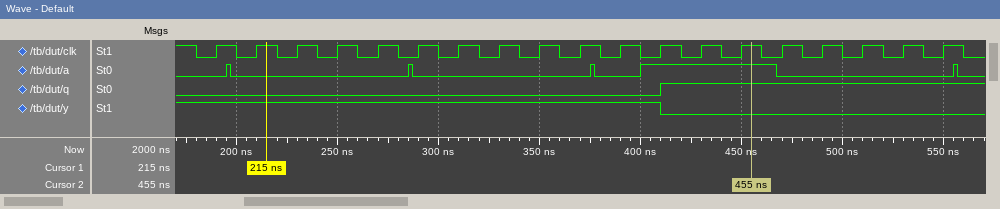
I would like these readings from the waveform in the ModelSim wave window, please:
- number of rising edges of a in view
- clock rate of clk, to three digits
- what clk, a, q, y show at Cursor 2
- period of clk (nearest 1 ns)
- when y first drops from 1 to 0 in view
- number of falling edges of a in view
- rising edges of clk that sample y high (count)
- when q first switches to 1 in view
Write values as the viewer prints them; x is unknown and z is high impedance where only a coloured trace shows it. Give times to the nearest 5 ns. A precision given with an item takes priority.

5
50.0 MHz
clk=1, a=1, q=1, y=0
20 ns
410 ns
5
12
410 ns
